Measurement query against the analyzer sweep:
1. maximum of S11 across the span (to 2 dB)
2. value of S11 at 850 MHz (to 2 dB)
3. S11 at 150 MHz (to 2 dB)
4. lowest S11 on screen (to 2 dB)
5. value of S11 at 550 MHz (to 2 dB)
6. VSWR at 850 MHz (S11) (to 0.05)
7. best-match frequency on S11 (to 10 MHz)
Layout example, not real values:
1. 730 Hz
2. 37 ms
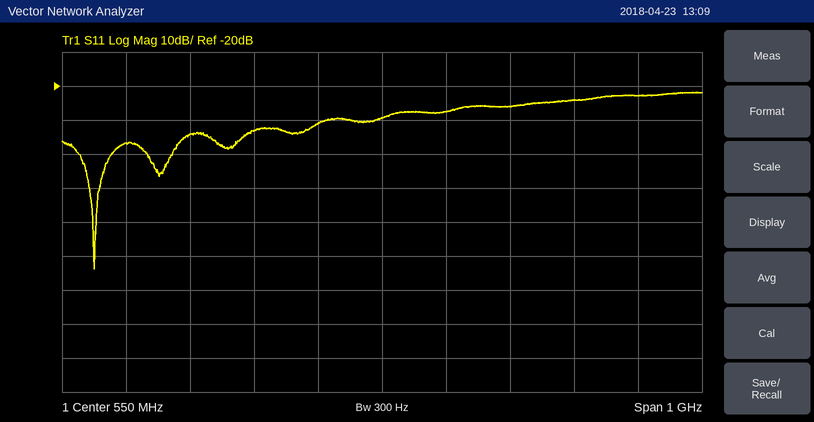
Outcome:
1. -22 dB
2. -24 dB
3. -36 dB
4. -74 dB
5. -30 dB
6. 1.15
7. 100 MHz
